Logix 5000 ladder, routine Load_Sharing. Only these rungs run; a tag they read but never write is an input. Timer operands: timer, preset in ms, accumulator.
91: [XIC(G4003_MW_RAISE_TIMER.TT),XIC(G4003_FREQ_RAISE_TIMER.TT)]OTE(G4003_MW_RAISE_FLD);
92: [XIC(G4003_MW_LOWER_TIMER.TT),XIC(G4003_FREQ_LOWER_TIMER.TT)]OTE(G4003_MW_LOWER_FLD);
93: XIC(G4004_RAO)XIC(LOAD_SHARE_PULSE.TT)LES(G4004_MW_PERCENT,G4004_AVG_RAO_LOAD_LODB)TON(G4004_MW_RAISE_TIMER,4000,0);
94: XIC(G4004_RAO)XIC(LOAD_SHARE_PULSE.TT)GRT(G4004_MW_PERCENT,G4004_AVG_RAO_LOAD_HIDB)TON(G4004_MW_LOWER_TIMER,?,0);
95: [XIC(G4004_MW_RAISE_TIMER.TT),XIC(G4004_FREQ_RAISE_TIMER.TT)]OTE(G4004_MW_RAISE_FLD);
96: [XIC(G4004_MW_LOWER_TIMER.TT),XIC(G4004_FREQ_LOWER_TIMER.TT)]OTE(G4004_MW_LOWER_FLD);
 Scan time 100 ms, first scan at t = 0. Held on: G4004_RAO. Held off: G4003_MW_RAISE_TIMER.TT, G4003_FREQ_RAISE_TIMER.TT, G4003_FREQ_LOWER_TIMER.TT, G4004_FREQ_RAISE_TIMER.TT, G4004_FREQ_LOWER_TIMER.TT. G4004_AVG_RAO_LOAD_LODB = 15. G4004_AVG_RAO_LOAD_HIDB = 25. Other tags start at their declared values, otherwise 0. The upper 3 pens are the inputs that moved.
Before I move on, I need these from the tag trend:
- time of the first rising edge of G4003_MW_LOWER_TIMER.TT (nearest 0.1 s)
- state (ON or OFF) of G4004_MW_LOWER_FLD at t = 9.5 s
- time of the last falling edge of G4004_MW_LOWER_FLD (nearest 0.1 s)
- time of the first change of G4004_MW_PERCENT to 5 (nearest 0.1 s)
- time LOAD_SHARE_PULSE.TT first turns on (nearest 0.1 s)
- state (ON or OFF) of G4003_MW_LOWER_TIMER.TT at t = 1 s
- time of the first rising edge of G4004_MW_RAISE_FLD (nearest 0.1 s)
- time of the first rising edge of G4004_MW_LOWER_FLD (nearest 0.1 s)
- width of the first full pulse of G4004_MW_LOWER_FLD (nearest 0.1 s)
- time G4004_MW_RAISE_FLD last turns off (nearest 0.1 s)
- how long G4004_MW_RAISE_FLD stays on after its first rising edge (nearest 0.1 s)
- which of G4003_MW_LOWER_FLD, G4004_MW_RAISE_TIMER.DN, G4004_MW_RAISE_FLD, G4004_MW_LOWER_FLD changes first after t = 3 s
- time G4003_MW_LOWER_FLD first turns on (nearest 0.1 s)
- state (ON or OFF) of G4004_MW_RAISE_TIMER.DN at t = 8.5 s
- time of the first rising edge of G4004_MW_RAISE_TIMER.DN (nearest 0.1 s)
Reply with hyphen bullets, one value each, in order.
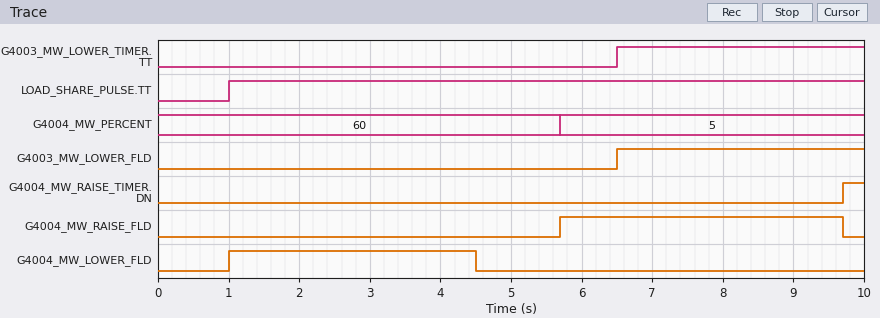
- 6.5 s
- OFF
- 4.5 s
- 5.7 s
- 1.0 s
- OFF
- 5.7 s
- 1.0 s
- 3.5 s
- 9.7 s
- 4.0 s
- G4004_MW_LOWER_FLD
- 6.5 s
- OFF
- 9.7 s
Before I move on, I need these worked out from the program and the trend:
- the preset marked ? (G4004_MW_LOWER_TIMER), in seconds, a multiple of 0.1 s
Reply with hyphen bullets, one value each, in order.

- 3.5 s
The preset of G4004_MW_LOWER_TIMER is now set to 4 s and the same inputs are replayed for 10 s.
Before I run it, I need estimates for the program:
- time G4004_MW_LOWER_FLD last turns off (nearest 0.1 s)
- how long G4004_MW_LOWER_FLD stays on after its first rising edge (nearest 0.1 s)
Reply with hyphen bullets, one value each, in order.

- 5.0 s
- 4.0 s
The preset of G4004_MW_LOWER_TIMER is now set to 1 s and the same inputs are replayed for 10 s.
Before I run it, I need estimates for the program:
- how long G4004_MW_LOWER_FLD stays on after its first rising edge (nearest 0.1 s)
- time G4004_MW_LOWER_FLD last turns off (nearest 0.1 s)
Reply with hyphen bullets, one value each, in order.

- 1.0 s
- 2.0 s
